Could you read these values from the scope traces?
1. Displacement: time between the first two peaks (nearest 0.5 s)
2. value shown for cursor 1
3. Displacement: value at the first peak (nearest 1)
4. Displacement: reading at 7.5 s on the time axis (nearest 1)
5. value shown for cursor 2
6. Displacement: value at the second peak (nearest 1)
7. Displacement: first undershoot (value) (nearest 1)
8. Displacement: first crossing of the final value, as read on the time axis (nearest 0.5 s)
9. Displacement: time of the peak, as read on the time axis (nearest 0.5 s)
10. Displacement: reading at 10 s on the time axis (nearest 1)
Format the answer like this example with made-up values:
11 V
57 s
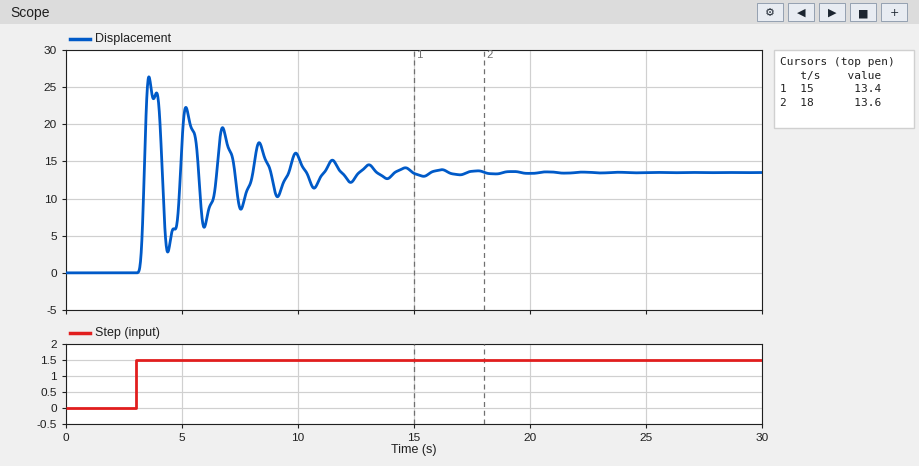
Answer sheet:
1.5 s
13.4
26
9
13.6
22
3
3.5 s
3.5 s
16
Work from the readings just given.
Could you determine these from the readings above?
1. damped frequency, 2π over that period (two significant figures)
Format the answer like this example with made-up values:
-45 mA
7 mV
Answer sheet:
4.2 rad/s
